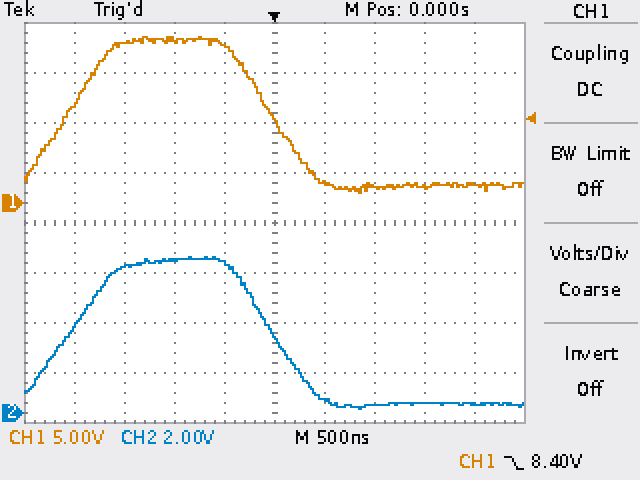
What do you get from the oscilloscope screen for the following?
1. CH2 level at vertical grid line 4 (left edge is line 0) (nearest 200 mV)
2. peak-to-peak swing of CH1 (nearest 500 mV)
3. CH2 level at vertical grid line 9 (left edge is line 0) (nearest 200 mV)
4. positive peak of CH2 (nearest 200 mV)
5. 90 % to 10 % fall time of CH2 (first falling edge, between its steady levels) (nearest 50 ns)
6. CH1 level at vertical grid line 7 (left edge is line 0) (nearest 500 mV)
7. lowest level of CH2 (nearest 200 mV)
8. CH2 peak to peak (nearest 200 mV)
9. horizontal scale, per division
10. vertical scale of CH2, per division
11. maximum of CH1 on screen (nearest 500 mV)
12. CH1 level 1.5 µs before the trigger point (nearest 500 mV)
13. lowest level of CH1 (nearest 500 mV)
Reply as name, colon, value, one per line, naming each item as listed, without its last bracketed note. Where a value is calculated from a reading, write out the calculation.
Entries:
CH2 level at vertical grid line 4 (left edge is line 0): 6.0 V
peak-to-peak swing of CH1: 16.5 V − (1.0 V) = 15.5 V
CH2 level at vertical grid line 9 (left edge is line 0): 400 mV
positive peak of CH2: 6.2 V
90 % to 10 % fall time of CH2 (first falling edge, between its steady levels): 750 ns
CH1 level at vertical grid line 7 (left edge is line 0): 1.5 V
lowest level of CH2: 200 mV
CH2 peak to peak: 6.2 V − (200 mV) = 6.0 V
horizontal scale, per division: 500 ns
vertical scale of CH2, per division: 2 V
maximum of CH1 on screen: 16.5 V
CH1 level 1.5 µs before the trigger point: 16.0 V
lowest level of CH1: 1.0 V
